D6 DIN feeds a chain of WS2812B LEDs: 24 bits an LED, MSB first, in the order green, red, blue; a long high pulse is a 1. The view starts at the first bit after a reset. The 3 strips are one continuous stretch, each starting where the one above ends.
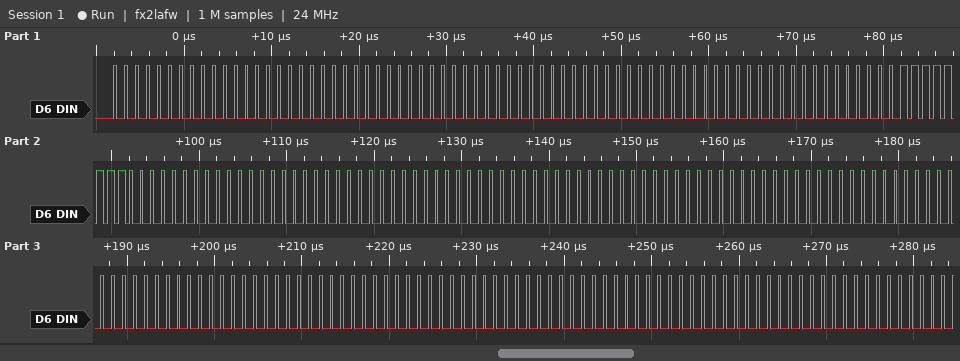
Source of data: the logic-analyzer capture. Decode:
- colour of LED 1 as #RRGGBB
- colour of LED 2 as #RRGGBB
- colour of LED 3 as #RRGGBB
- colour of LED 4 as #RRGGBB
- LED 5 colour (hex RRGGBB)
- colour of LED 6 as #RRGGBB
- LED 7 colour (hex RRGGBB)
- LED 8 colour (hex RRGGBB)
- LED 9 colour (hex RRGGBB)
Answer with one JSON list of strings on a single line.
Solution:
["#000000", "#000000", "#000000", "#00FF00", "#000000", "#000000", "#000000", "#000000", "#000000"]
